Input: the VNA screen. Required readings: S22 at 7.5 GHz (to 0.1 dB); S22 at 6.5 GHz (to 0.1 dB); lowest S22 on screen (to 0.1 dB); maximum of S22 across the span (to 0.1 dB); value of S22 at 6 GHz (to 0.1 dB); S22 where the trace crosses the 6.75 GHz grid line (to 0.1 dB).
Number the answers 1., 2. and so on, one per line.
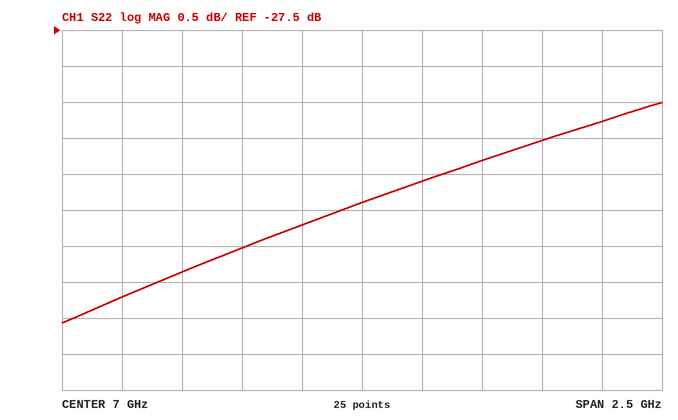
1. -29.3 dB
2. -30.5 dB
3. -31.6 dB
4. -28.5 dB
5. -31.2 dB
6. -30.2 dB
